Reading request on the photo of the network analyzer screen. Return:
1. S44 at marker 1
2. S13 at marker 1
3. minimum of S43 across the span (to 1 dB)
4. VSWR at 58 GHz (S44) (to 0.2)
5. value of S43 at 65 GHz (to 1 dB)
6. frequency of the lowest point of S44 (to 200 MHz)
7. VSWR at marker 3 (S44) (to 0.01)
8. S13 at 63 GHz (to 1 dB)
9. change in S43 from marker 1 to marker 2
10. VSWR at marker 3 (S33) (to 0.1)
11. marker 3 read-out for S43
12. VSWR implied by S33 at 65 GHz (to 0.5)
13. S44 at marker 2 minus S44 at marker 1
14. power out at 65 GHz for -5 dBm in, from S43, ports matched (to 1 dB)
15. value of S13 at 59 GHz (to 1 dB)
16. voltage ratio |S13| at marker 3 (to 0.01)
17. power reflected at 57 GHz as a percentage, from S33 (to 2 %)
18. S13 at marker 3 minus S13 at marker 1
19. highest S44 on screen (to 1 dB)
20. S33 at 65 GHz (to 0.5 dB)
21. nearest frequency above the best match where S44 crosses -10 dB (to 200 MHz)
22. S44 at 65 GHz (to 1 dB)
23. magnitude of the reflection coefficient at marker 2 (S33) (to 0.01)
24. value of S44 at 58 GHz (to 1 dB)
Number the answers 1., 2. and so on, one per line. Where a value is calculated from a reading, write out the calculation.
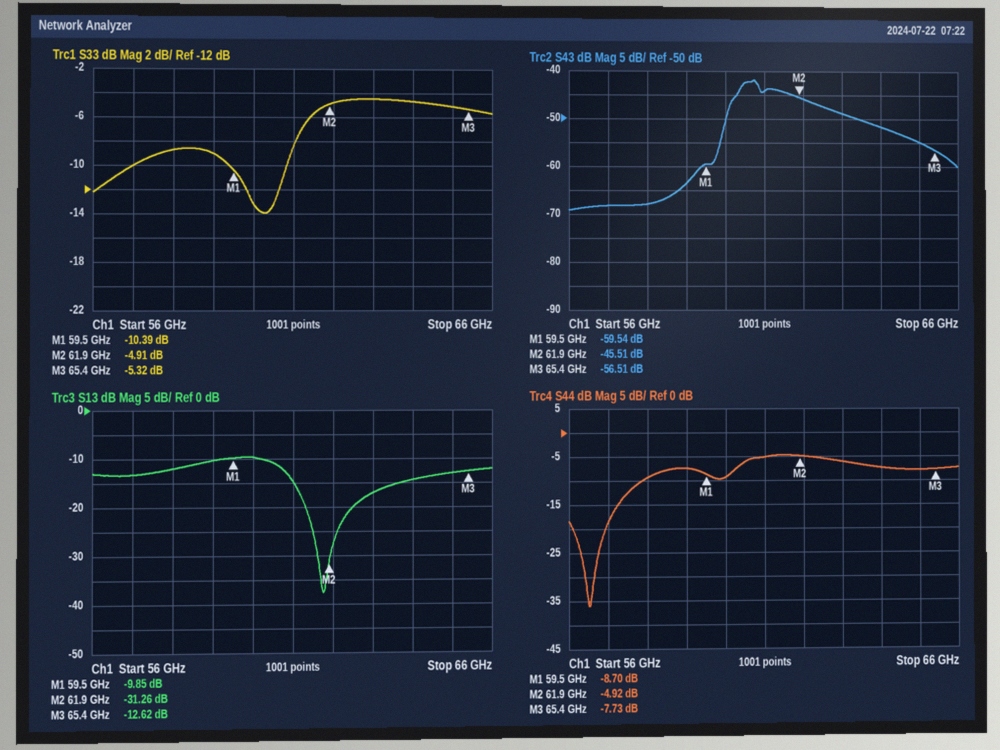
1. -8.70 dB
2. -9.85 dB
3. -69 dB
4. |Γ| = 10^(-9/20) = 0.3548; VSWR = (1 + 0.3548)/(1 − 0.3548) ≈ 2.10, so 2.0 to the nearest 0.2
5. -55 dB
6. 56.6 GHz
7. (1 + 0.4107)/(1 − 0.4107) ≈ 2.39
8. -17 dB
9. -45.51 − (-59.54) = 14.03 dB
10. (1 + 0.5420)/(1 − 0.5420) ≈ 3.4
11. -56.51 dB
12. |Γ| = 10^(-5/20) = 0.5623; VSWR = (1 + 0.5623)/(1 − 0.5623) ≈ 3.57, so 3.5 to the nearest 0.5
13. -4.92 − (-8.7) = 3.78 dB
14. -5 dBm + (-55 dB) = -60 dBm
15. -10 dB
16. 10^(-12.62/20) ≈ 0.23
17. 10^(-10/10) ≈ 10 %
18. -12.62 − (-9.85) = -2.77 dB
19. -5 dB
20. -5.0 dB
21. 57.8 GHz
22. -8 dB
23. 10^(-4.91/20) ≈ 0.57
24. -9 dB
